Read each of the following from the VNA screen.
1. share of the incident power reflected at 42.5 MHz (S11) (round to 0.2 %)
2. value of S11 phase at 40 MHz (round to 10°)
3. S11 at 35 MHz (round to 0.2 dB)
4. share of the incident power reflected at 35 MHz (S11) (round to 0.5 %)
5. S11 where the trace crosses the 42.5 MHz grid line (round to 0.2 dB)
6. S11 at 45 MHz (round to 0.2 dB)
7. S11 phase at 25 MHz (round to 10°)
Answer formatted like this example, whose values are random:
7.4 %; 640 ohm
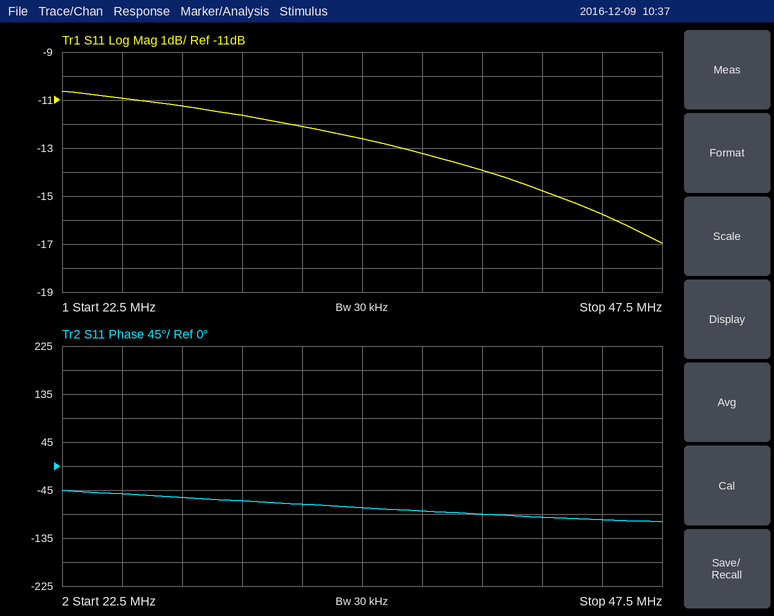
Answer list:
3.4 %; -90°; -12.6 dB; 5.5 %; -14.8 dB; -15.8 dB; -50°
